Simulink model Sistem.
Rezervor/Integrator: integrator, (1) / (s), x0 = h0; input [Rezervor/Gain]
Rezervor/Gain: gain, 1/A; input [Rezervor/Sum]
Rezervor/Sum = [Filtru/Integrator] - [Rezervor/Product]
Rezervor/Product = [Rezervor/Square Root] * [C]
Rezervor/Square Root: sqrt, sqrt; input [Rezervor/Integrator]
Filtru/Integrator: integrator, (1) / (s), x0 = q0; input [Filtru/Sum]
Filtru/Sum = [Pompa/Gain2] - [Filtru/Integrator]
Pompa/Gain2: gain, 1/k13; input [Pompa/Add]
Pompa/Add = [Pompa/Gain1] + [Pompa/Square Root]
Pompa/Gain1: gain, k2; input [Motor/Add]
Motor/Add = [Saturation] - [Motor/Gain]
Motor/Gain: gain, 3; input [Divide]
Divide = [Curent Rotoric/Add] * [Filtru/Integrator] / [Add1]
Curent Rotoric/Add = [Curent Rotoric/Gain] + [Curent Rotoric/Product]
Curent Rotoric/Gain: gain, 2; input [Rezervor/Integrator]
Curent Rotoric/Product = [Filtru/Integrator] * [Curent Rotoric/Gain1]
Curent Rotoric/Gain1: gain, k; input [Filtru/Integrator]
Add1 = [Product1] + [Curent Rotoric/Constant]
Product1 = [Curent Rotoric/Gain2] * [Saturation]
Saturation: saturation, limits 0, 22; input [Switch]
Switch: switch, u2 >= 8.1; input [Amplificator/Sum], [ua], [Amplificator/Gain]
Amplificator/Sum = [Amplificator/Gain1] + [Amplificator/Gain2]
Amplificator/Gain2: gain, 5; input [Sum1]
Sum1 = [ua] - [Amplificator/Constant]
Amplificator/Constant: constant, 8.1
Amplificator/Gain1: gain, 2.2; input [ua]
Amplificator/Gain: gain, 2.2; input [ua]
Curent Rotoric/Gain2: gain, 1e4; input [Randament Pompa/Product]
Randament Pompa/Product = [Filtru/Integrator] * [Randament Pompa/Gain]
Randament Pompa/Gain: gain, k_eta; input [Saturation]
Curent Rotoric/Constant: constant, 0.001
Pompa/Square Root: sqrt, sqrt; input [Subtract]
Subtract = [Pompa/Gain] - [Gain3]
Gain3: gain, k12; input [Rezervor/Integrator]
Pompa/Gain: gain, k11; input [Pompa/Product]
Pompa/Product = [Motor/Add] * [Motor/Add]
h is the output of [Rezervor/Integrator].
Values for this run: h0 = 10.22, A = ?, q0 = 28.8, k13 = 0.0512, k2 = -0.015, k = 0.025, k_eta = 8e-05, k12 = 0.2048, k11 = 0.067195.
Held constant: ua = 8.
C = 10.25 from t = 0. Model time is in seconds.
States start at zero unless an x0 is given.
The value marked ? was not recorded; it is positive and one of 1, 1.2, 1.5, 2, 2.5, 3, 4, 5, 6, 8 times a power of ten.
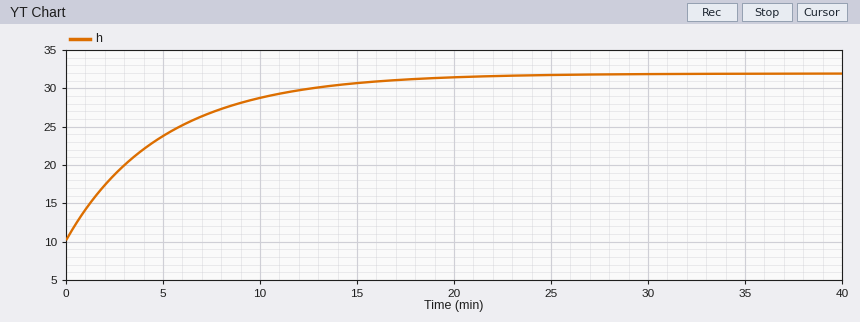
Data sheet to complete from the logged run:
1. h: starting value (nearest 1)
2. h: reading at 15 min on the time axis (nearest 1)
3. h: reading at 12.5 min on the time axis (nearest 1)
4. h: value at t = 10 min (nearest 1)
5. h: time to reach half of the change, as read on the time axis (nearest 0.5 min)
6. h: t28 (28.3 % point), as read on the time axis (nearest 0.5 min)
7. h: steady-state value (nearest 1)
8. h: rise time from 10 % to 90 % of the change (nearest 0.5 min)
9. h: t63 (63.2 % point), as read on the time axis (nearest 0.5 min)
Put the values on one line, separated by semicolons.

10; 31; 30; 29; 3.5 min; 1.5 min; 32; 11.5 min; 5.0 min
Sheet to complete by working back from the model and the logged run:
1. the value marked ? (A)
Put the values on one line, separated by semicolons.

500
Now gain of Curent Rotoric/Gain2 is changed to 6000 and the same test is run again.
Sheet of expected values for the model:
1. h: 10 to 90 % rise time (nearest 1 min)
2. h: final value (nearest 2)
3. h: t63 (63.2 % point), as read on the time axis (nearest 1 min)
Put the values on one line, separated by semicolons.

11 min; 28; 5 min
